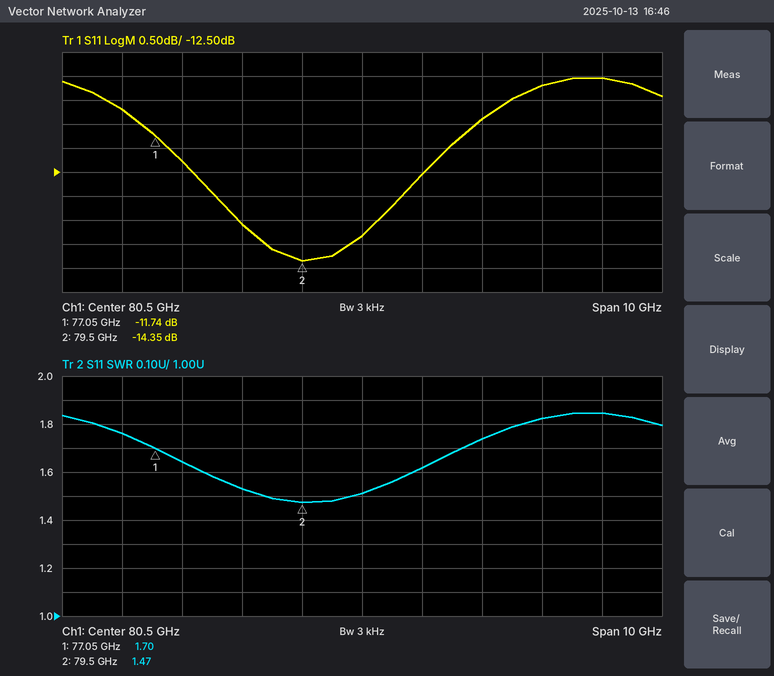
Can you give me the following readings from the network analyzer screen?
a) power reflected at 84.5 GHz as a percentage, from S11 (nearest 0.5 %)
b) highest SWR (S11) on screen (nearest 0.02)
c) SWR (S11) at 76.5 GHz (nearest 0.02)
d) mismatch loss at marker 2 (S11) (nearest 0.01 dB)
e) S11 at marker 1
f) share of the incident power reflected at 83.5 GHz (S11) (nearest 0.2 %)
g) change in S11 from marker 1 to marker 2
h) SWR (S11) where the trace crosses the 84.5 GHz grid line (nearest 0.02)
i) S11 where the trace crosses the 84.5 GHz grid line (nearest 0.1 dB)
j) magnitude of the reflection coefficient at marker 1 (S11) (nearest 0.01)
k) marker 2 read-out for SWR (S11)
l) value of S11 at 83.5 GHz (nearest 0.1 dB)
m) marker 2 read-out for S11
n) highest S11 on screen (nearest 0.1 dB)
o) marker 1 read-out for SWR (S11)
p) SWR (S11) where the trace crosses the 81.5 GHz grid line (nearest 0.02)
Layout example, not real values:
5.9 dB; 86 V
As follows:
9.0 %; 1.84; 1.76; 0.16 dB; -11.74 dB; 8.6 %; -2.61 dB; 1.84; -10.5 dB; 0.26; 1.47; -10.7 dB; -14.35 dB; -10.5 dB; 1.70; 1.62
